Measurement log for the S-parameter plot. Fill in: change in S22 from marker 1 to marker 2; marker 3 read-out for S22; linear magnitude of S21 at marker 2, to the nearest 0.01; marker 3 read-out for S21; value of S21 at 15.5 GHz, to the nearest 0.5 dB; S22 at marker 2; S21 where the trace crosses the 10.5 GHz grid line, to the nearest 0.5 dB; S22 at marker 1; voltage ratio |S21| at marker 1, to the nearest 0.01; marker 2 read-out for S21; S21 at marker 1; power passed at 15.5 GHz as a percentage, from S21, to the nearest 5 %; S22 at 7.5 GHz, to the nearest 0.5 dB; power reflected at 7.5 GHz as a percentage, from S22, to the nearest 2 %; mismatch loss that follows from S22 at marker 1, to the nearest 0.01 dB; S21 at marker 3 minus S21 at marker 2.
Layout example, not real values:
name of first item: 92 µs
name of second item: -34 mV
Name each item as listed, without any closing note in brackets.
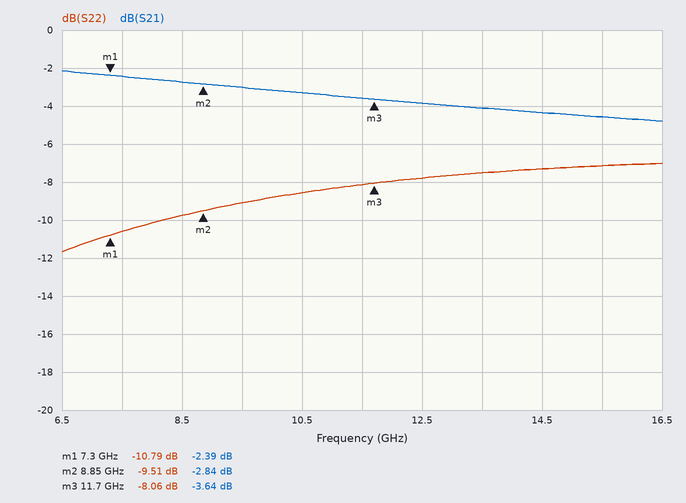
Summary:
change in S22 from marker 1 to marker 2: 1.28 dB
marker 3 read-out for S22: -8.06 dB
linear magnitude of S21 at marker 2, to the nearest 0.01: 0.72
marker 3 read-out for S21: -3.64 dB
value of S21 at 15.5 GHz, to the nearest 0.5 dB: -4.5 dB
S22 at marker 2: -9.51 dB
S21 where the trace crosses the 10.5 GHz grid line, to the nearest 0.5 dB: -3.5 dB
S22 at marker 1: -10.79 dB
voltage ratio |S21| at marker 1, to the nearest 0.01: 0.76
marker 2 read-out for S21: -2.84 dB
S21 at marker 1: -2.39 dB
power passed at 15.5 GHz as a percentage, from S21, to the nearest 5 %: 35 %
S22 at 7.5 GHz, to the nearest 0.5 dB: -10.5 dB
power reflected at 7.5 GHz as a percentage, from S22, to the nearest 2 %: 8 %
mismatch loss that follows from S22 at marker 1, to the nearest 0.01 dB: 0.38 dB
S21 at marker 3 minus S21 at marker 2: -0.80 dB
